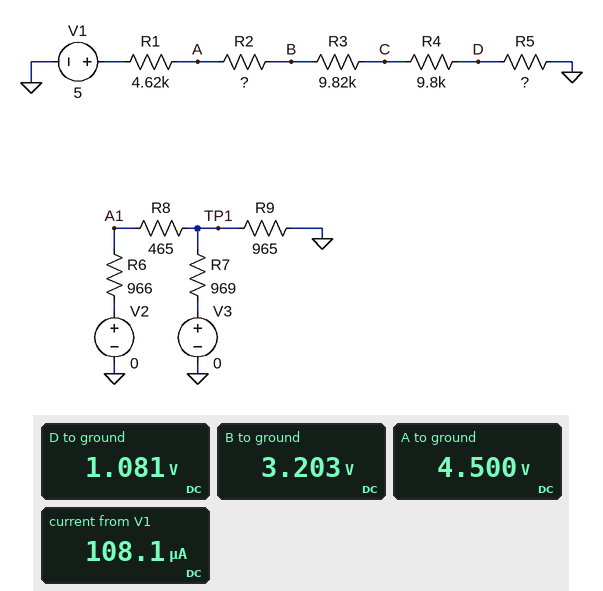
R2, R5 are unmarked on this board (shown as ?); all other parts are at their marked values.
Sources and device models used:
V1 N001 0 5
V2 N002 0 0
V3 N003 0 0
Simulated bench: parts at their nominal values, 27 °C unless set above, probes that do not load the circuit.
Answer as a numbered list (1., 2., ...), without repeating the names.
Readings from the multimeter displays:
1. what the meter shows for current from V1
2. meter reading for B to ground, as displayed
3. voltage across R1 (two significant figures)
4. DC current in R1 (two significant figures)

1. 108.1 µA
2. 3.203 V
3. 500 mV
4. 110 µA
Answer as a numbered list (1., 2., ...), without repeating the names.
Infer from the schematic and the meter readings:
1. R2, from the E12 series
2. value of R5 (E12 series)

1. 12 kΩ
2. 10 kΩ
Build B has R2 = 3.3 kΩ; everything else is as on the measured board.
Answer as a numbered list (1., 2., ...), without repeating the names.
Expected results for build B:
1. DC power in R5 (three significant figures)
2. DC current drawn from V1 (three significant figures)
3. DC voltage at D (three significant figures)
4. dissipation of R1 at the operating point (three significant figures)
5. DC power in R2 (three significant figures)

1. 177 µW
2. 133 µA
3. 1.33 V
4. 82.0 µW
5. 58.5 µW
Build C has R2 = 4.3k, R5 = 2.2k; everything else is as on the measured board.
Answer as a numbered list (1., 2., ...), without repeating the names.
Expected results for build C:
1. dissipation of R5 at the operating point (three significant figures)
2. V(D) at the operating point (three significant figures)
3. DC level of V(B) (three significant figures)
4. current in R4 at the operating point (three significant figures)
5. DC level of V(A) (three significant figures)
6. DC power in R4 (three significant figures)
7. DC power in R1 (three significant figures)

1. 58.2 µW
2. 358 mV
3. 3.55 V
4. 163 µA
5. 4.25 V
6. 259 µW
7. 122 µW
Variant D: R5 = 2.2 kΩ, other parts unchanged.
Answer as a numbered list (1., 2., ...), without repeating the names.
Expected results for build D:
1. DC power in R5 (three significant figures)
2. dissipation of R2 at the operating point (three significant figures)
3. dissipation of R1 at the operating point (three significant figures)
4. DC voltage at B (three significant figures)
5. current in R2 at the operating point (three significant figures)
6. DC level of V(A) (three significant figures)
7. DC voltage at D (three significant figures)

1. 37.2 µW
2. 203 µW
3. 78.2 µW
4. 2.84 V
5. 130 µA
6. 4.40 V
7. 286 mV
